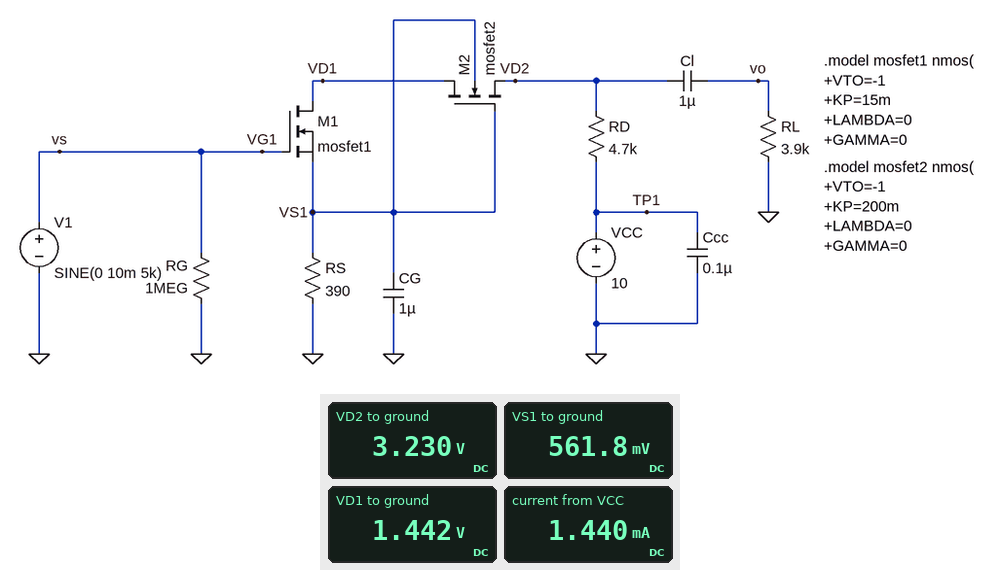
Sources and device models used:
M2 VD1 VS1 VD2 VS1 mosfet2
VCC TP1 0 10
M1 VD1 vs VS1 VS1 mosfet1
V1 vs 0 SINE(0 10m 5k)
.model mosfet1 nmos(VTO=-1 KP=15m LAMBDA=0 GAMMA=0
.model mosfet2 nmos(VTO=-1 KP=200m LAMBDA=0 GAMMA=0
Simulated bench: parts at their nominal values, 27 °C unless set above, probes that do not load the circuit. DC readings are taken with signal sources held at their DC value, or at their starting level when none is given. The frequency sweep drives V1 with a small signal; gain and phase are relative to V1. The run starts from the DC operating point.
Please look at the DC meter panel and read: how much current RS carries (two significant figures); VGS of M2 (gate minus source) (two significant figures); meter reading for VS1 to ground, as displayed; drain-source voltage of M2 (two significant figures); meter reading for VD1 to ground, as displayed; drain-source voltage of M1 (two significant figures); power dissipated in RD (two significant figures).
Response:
1.4 mA
-2.7 V
561.8 mV
-1.8 V
1.442 V
880 mV
9.8 mW
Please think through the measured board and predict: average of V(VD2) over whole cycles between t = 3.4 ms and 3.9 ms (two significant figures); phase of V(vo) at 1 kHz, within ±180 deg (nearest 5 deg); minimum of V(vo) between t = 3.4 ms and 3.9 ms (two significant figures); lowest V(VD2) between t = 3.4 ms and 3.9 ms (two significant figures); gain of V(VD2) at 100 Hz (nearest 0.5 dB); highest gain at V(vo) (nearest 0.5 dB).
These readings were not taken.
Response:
3.2 V
-145 deg
-140 mV
3.1 V
12.5 dB
23.0 dB
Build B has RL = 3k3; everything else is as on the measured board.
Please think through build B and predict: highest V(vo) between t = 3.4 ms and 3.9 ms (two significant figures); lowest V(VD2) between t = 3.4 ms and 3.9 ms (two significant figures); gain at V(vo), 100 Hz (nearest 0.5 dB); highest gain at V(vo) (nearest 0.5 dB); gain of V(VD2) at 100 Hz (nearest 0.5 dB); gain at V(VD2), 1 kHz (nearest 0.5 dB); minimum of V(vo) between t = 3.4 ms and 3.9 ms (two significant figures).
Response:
120 mV
3.1 V
11.0 dB
22.0 dB
12.0 dB
18.0 dB
-120 mV
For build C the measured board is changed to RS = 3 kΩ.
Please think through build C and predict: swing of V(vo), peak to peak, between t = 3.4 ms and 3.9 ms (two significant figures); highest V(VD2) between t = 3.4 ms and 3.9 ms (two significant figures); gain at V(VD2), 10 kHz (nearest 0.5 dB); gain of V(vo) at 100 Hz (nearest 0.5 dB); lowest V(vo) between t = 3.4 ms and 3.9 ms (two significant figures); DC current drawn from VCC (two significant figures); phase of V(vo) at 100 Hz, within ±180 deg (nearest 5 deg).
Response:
120 mV
8.8 V
15.5 dB
2.5 dB
-61 mV
270 µA
-120 deg
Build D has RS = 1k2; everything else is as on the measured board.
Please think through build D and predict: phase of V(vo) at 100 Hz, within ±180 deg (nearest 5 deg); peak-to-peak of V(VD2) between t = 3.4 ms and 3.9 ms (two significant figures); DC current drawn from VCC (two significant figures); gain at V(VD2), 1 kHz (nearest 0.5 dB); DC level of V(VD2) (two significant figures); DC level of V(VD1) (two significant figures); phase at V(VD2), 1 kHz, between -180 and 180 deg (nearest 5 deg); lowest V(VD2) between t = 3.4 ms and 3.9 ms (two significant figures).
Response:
-140 deg
180 mV
600 µA
17.0 dB
7.2 V
1.6 V
-150 deg
7.1 V
